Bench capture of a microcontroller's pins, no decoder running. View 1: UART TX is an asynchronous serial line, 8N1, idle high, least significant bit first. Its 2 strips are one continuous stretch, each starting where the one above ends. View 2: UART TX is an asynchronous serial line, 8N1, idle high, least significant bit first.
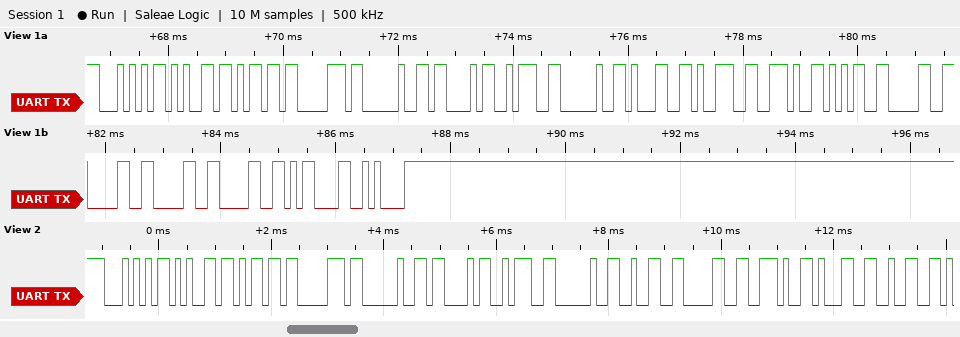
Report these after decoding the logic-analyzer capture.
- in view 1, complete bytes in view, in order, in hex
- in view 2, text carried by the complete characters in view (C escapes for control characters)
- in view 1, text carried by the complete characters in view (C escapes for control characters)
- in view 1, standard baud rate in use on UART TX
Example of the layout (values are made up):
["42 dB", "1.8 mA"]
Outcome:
["54 65 6D 70 20 43 3A 20 31 39 2E 35 30 30 30 30 0D 0A", "\"Temp C: 20.12\"", "\"Temp C: 19.50000\\r\\n\"", "9600 baud"]
